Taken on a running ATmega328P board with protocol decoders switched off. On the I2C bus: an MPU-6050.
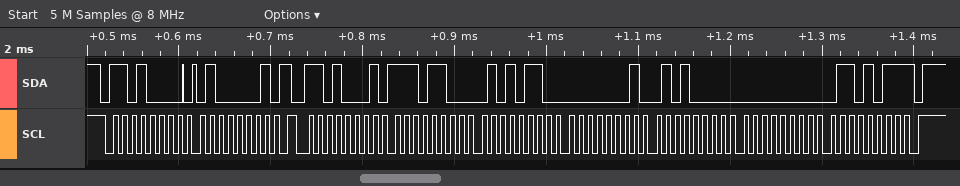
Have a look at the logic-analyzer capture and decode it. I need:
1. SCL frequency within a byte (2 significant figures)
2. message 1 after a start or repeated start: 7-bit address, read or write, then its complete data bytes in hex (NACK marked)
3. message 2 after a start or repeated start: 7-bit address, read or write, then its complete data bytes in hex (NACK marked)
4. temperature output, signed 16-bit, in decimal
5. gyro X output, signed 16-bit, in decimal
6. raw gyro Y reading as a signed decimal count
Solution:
100 kHz
0x68 write: 41
0x68 read: EC 56 01 50 00 6B NACK
-5034
336
107
